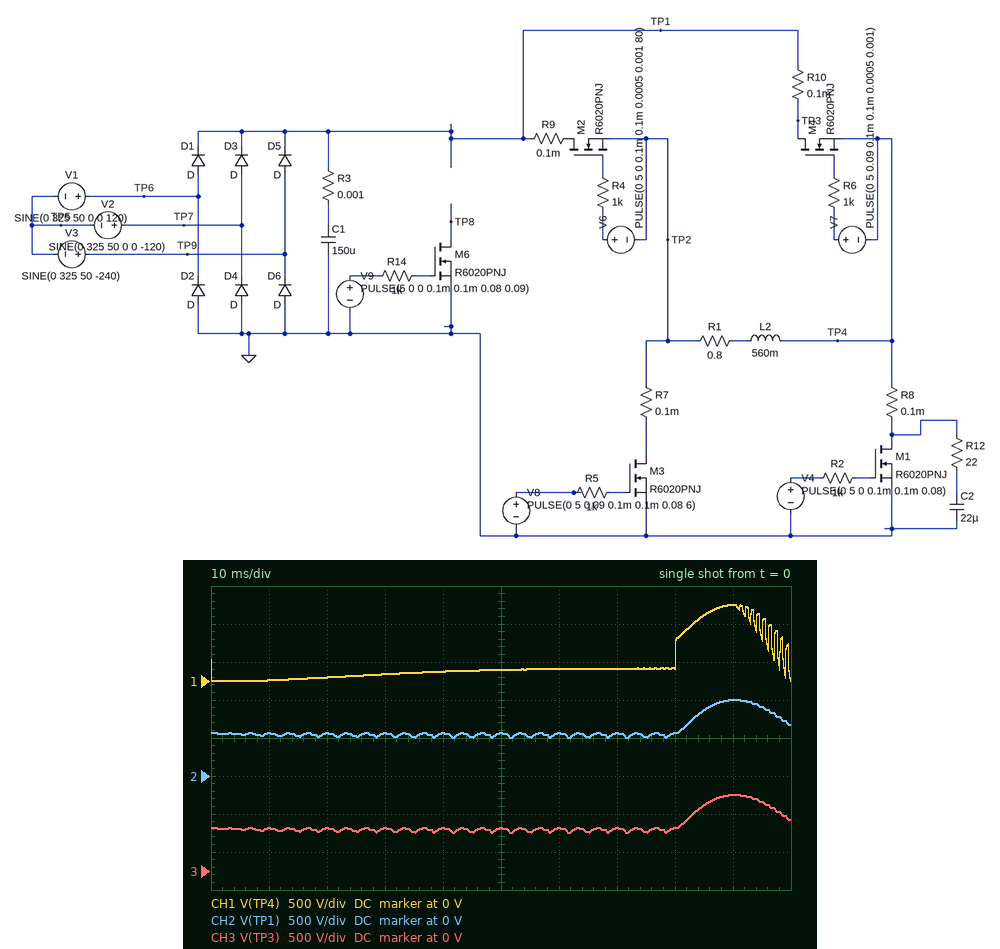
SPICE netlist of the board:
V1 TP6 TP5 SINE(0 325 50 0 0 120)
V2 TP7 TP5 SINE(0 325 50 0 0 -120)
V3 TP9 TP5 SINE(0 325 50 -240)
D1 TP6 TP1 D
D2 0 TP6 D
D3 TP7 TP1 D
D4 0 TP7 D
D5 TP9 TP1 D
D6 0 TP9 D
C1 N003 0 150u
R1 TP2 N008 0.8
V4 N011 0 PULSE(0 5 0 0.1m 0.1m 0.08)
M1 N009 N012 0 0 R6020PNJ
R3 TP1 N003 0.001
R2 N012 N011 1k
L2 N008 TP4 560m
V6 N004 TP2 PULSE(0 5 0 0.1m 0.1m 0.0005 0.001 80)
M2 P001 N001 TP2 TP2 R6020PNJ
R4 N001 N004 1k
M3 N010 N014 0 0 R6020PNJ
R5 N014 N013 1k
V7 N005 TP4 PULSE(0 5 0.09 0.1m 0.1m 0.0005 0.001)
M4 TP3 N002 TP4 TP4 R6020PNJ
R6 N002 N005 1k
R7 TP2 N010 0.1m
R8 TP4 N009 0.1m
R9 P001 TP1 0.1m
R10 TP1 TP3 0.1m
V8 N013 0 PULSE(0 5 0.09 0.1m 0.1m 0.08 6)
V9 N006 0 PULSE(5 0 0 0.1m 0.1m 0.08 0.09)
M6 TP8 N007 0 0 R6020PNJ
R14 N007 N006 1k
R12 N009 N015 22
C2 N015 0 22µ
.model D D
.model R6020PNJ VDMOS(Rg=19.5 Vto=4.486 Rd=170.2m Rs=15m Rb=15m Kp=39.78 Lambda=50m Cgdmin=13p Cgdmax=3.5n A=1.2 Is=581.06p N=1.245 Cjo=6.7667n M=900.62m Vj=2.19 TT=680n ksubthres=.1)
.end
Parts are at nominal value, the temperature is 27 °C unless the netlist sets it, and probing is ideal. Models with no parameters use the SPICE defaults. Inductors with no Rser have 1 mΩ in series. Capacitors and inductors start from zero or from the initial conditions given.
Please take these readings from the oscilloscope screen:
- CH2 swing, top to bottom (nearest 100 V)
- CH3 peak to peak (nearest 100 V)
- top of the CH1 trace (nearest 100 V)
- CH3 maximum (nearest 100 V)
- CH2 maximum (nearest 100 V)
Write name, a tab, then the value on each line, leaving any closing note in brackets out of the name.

CH2 swing, top to bottom	500 V
CH3 peak to peak	500 V
top of the CH1 trace	1.0 kV
CH3 maximum	1.0 kV
CH2 maximum	1.0 kV
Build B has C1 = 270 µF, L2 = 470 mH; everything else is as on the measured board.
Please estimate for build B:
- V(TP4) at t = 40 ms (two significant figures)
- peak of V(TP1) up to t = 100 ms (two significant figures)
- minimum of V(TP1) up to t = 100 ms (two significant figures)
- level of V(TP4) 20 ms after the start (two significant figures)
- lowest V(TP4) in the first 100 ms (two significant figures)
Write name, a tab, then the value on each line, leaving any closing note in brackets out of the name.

V(TP4) at t = 40 ms	140 V
peak of V(TP1) up to t = 100 ms	810 V
minimum of V(TP1) up to t = 100 ms	510 V
level of V(TP4) 20 ms after the start	63 V
lowest V(TP4) in the first 100 ms	-780 mV
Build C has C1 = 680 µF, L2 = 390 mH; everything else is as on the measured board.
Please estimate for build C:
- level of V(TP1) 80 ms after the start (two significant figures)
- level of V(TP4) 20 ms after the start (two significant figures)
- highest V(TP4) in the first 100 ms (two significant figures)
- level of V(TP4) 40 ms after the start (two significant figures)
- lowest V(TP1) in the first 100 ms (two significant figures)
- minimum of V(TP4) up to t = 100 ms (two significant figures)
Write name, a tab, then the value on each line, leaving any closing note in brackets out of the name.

level of V(TP1) 80 ms after the start	560 V
level of V(TP4) 20 ms after the start	85 V
highest V(TP4) in the first 100 ms	660 V
level of V(TP4) 40 ms after the start	160 V
lowest V(TP1) in the first 100 ms	530 V
minimum of V(TP4) up to t = 100 ms	-790 mV
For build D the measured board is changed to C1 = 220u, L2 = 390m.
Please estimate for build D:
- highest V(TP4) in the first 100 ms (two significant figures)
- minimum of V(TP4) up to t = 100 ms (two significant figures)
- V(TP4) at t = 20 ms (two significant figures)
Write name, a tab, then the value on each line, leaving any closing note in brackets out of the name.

highest V(TP4) in the first 100 ms	800 V
minimum of V(TP4) up to t = 100 ms	-830 mV
V(TP4) at t = 20 ms	83 V
